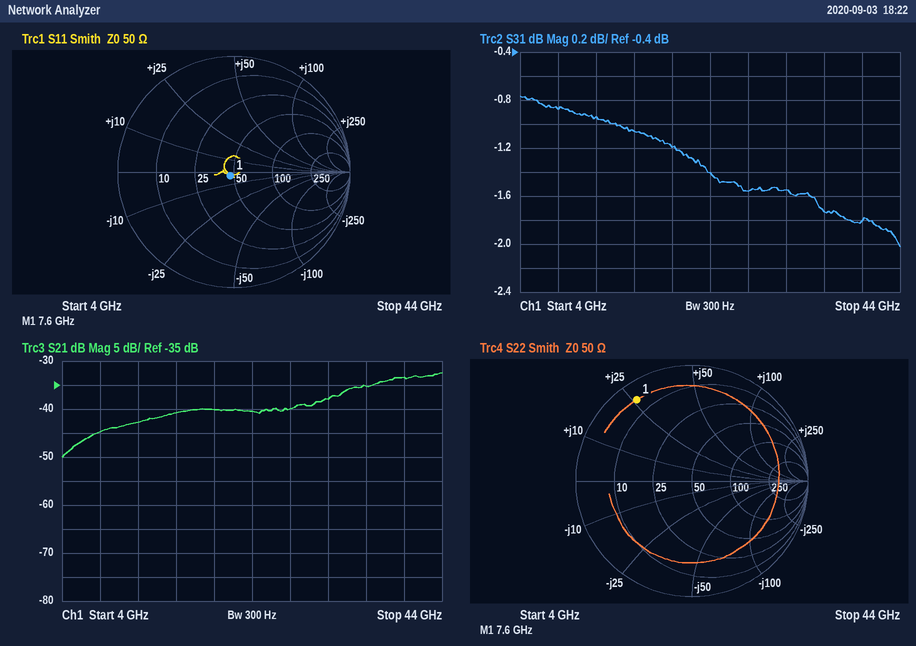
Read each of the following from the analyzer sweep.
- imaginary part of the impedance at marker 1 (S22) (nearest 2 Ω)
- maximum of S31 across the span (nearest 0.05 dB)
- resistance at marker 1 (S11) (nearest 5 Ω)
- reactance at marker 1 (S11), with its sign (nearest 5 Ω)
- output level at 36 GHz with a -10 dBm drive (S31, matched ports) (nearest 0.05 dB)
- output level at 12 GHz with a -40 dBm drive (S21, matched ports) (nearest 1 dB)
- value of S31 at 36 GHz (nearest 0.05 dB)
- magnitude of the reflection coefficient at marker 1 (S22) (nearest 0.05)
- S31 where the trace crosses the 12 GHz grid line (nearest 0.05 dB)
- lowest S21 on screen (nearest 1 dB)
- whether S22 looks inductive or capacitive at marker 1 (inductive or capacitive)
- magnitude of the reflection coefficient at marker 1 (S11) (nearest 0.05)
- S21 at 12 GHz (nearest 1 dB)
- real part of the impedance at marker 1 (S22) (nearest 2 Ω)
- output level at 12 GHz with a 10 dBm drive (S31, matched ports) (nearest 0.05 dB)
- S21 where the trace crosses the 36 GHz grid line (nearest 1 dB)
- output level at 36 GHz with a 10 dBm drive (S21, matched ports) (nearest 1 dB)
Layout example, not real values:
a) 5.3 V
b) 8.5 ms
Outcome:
a) +26 Ω
b) -0.75 dB
c) 45 Ω
d) -5 Ω
e) -11.75 dBm
f) -83 dBm
g) -1.75 dB
h) 0.85
i) -0.95 dB
j) -50 dB
k) inductive
l) 0.05
m) -43 dB
n) 6 Ω
o) 9.05 dBm
p) -35 dB
q) -25 dBm
